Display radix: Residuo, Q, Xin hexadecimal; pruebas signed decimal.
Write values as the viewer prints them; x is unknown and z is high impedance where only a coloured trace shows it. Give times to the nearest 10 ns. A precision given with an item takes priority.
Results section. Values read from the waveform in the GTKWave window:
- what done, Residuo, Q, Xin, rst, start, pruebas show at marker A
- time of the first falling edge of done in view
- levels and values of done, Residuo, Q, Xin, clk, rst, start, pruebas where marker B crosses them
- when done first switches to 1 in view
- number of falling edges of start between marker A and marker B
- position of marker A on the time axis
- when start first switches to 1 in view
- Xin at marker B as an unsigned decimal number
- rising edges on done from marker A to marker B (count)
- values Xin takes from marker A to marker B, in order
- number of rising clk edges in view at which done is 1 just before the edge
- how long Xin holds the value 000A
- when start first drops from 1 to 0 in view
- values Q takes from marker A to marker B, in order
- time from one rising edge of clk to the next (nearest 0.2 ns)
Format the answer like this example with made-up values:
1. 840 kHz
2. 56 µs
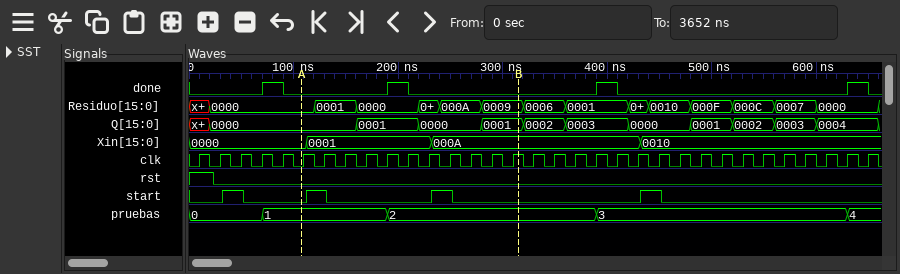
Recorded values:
1. done=0, Residuo=0000, Q=0000, Xin=0000, rst=0, start=0, pruebas=1
2. 90 ns
3. done=0, Residuo=0009, Q=0001, Xin=000A, clk=1, rst=0, start=0, pruebas=2
4. 70 ns
5. 2
6. 110 ns
7. 30 ns
8. 10
9. 1
10. 0000, 0001, 000A
11. 4
12. 200 ns
13. 50 ns
14. 0000, 0001, 0000, 0001
15. 20 ns
